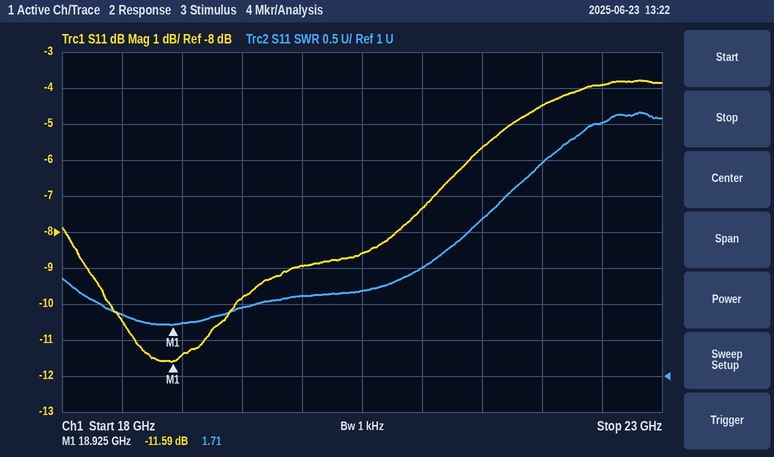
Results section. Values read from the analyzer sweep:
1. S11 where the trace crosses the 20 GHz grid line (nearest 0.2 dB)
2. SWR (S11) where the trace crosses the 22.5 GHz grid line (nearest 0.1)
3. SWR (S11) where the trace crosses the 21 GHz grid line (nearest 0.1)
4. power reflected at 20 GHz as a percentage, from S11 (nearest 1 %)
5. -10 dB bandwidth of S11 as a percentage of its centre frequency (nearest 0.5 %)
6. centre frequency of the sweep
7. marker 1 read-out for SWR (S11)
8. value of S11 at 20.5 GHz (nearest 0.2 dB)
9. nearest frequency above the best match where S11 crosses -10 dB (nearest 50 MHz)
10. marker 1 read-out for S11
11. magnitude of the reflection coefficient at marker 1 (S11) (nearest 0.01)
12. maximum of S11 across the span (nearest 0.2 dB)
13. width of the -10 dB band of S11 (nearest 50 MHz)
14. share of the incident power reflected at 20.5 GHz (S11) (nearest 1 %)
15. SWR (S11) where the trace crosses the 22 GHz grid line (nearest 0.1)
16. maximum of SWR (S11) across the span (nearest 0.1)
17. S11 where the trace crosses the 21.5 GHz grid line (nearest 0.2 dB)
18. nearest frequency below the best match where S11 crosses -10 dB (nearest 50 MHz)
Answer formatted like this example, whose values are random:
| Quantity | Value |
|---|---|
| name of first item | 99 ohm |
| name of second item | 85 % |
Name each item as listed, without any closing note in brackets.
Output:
| Quantity | Value |
|---|---|
| S11 where the trace crosses the 20 GHz grid line | -9.0 dB |
| SWR (S11) where the trace crosses the 22.5 GHz grid line | 4.5 |
| SWR (S11) where the trace crosses the 21 GHz grid line | 2.5 |
| power reflected at 20 GHz as a percentage, from S11 | 13 % |
| -10 dB bandwidth of S11 as a percentage of its centre frequency | 5.5 % |
| centre frequency of the sweep | 20.5 GHz |
| marker 1 read-out for SWR | 1.71 |
| value of S11 at 20.5 GHz | -8.6 dB |
| nearest frequency above the best match where S11 crosses -10 dB | 19.45 GHz |
| marker 1 read-out for S11 | -11.59 dB |
| magnitude of the reflection coefficient at marker 1 (S11) | 0.26 |
| maximum of S11 across the span | -3.8 dB |
| width of the -10 dB band of S11 | 1.05 GHz |
| share of the incident power reflected at 20.5 GHz (S11) | 14 % |
| SWR (S11) where the trace crosses the 22 GHz grid line | 4.0 |
| maximum of SWR (S11) across the span | 4.7 |
| S11 where the trace crosses the 21.5 GHz grid line | -5.6 dB |
| nearest frequency below the best match where S11 crosses -10 dB | 18.40 GHz |
